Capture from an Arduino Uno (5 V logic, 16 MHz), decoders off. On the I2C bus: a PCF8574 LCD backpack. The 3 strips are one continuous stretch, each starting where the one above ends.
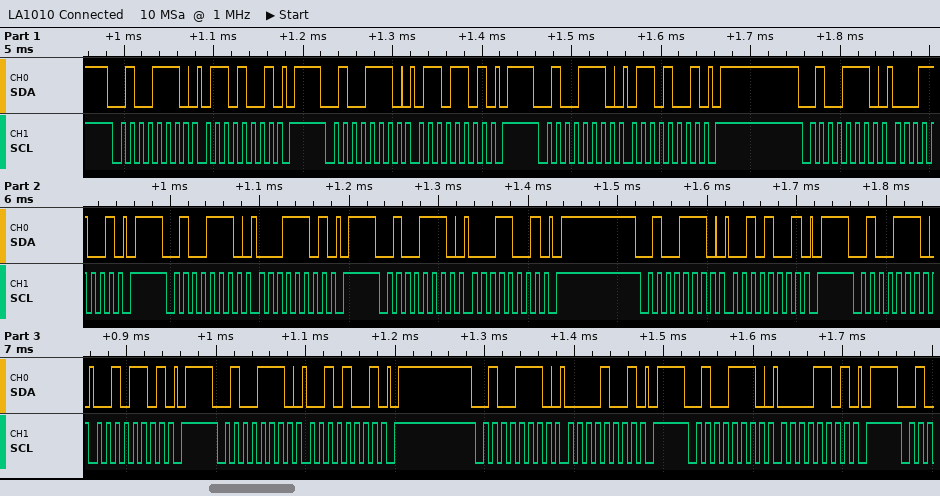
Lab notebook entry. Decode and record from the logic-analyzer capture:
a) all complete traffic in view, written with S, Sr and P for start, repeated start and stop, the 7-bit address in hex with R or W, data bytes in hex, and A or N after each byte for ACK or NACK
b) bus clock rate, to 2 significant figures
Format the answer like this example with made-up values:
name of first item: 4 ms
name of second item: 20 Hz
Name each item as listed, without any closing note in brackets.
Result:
all complete traffic in view, written with S, Sr and P for start, repeated start and stop, the 7-bit address in hex with R or W, data bytes in hex, and A or N after each byte for ACK or NACK: S 27W A 69 A P S 27W A 6D A P S 27W A 69 A P S 27W A 19 A P S 27W A 1D A P S 27W A 19 A P S 27W A 29 A P S 27W A 2D A P S 27W A 29 A P S 27W A 09 A P S 27W A 0D A P
bus clock rate, to 2 significant figures: 100 kHz
